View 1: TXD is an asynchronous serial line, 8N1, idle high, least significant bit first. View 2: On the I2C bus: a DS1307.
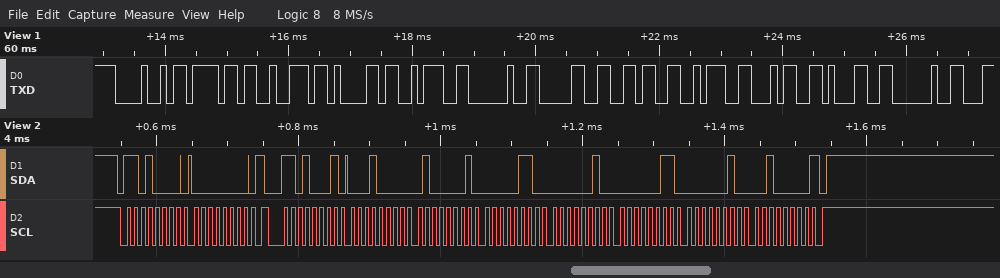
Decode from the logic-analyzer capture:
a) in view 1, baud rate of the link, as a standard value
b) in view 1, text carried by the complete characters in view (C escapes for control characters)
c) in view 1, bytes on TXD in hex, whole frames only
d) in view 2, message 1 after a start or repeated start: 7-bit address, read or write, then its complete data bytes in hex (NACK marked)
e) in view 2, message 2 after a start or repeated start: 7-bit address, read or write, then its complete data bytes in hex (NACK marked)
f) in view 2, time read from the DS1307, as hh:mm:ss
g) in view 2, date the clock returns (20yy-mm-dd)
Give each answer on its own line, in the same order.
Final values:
9600 baud
"Hora: 06:41 "
48 6F 72 61 3A 20 30 36 3A 34 31 20
0x68 write: 00
0x68 read: 10 41 06 02 03 02 20 NACK
06:41:10
2020-02-03
